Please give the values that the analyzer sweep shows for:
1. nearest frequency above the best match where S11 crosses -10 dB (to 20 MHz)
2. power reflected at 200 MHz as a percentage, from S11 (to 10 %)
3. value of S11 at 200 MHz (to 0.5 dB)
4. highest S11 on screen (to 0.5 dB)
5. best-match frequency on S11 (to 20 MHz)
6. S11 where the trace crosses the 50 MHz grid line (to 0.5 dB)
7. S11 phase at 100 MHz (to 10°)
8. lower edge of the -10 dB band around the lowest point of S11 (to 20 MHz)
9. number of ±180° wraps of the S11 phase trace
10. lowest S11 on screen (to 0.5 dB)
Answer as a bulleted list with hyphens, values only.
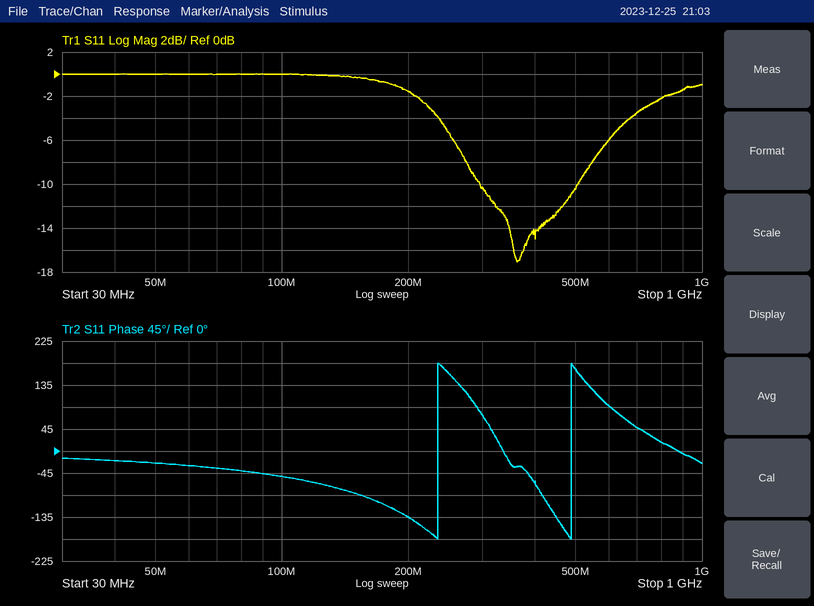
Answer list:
- 500 MHz
- 70 %
- -1.5 dB
- 0.0 dB
- 360 MHz
- 0.0 dB
- -50°
- 300 MHz
- 2
- -17.0 dB
